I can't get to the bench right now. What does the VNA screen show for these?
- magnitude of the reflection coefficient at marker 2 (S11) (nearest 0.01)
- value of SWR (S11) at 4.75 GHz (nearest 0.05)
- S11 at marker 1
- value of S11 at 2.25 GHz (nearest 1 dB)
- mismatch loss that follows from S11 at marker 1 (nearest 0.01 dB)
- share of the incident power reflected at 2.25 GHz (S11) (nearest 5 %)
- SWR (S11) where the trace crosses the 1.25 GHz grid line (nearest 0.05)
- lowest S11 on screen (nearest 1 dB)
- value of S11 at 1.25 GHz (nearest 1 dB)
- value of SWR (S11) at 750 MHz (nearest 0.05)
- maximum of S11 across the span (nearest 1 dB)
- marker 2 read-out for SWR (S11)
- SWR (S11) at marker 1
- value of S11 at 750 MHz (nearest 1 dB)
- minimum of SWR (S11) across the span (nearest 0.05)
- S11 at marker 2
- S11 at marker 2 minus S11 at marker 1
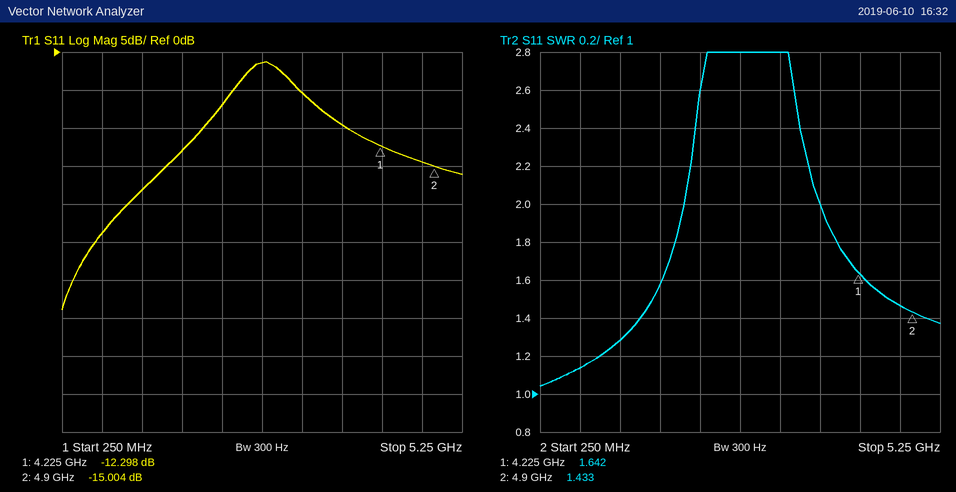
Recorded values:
0.18
1.45
-12.298 dB
-7 dB
0.26 dB
20 %
1.30
-34 dB
-18 dB
1.15
-1 dB
1.433
1.642
-24 dB
1.05
-15.004 dB
-2.706 dB
